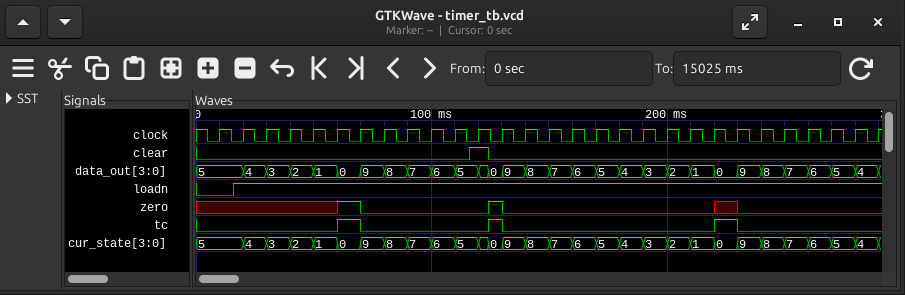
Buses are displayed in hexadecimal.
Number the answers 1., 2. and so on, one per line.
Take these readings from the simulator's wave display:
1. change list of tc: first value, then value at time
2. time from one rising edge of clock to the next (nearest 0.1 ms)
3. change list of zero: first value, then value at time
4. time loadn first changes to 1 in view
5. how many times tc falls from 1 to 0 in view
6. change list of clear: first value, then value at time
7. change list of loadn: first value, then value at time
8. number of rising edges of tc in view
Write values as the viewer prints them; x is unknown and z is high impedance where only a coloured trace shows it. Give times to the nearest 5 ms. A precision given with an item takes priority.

1. 0, 1 at 60 ms, 0 at 70 ms, 1 at 125 ms, 0 at 130 ms, 1 at 220 ms, 0 at 230 ms
2. 10 ms
3. x, 1 at 60 ms, 0 at 70 ms, 1 at 125 ms, 0 at 130 ms, x at 220 ms, 0 at 230 ms
4. 15 ms
5. 3
6. 0, 1 at 115 ms, 0 at 125 ms
7. 0, 1 at 15 ms
8. 3
